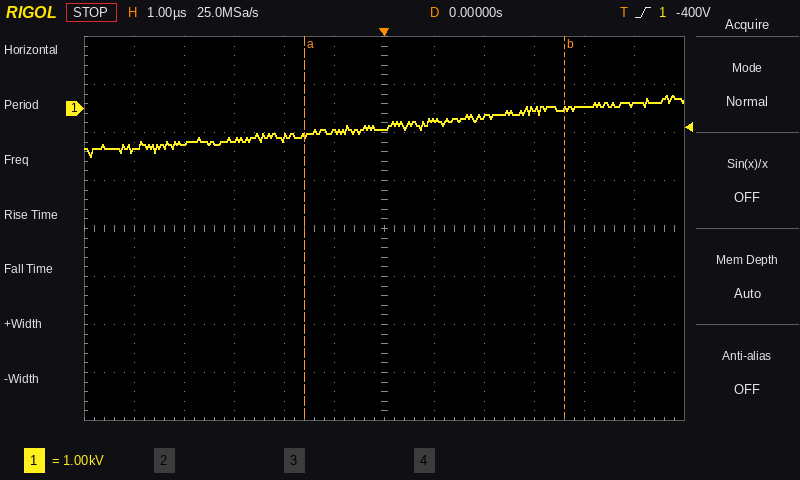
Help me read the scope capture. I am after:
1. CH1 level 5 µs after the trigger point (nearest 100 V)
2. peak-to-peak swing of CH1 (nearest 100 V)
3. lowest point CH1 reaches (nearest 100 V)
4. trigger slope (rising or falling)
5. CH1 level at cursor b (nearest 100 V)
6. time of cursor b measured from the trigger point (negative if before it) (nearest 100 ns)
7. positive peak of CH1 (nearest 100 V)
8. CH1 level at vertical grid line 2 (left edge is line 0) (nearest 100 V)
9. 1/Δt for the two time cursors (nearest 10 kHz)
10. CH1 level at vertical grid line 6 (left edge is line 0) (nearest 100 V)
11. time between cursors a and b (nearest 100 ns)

100 V
1.3 kV
-1.0 kV
rising
0.0 kV
+3.6 µs
300 V
-700 V
190 kHz
-400 V
5.2 µs
